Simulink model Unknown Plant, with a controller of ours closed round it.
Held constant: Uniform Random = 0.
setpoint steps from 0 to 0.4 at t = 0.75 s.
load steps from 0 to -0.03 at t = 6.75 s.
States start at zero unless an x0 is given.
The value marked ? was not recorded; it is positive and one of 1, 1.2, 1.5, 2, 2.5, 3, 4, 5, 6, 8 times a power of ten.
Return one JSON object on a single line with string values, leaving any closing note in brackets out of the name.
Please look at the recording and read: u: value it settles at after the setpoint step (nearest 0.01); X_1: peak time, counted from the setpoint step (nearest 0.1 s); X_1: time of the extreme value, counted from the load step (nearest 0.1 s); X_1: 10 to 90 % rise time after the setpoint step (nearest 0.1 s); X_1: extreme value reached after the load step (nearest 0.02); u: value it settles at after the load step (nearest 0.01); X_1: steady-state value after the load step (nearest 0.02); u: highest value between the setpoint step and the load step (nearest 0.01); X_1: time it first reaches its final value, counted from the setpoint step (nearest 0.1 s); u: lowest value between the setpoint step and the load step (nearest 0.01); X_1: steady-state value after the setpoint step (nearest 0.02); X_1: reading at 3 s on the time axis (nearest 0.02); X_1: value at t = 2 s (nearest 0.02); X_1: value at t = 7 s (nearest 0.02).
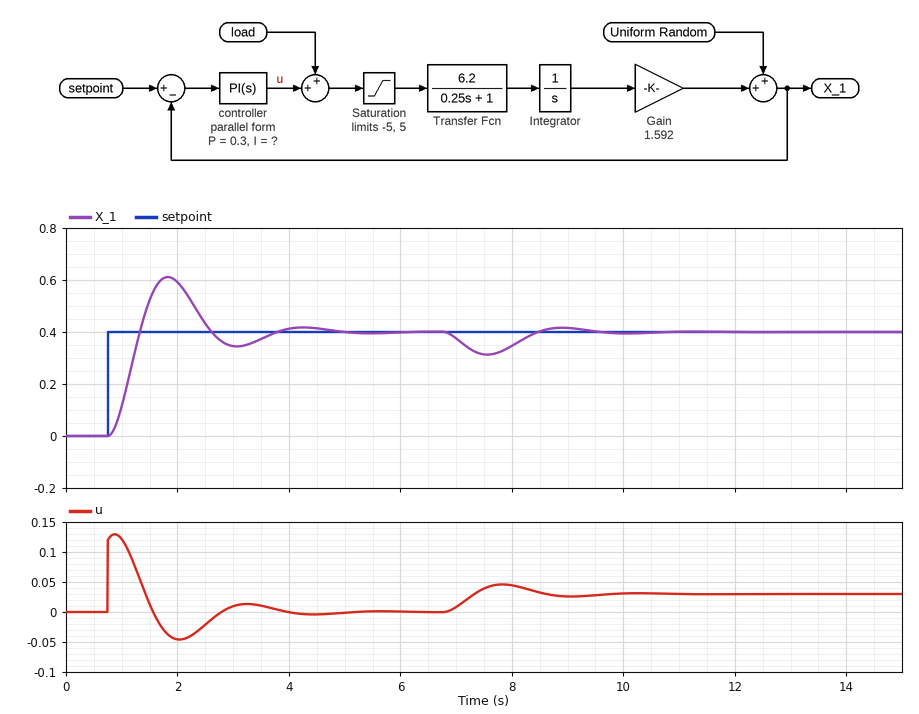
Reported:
{"u: value it settles at after the setpoint step": "0.00", "X_1: peak time, counted from the setpoint step": "1.1 s", "X_1: time of the extreme value, counted from the load step": "0.8 s", "X_1: 10 to 90 % rise time after the setpoint step": "0.4 s", "X_1: extreme value reached after the load step": "0.32", "u: value it settles at after the load step": "0.03", "X_1: steady-state value after the load step": "0.40", "u: highest value between the setpoint step and the load step": "0.13", "X_1: time it first reaches its final value, counted from the setpoint step": "0.6 s", "u: lowest value between the setpoint step and the load step": "-0.05", "X_1: steady-state value after the setpoint step": "0.40", "X_1: reading at 3 s on the time axis": "0.34", "X_1: value at t = 2 s": "0.60", "X_1: value at t = 7 s": "0.38"}
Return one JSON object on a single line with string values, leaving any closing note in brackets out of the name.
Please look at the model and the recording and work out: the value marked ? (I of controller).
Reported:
{"the value marked ?": "0.4"}
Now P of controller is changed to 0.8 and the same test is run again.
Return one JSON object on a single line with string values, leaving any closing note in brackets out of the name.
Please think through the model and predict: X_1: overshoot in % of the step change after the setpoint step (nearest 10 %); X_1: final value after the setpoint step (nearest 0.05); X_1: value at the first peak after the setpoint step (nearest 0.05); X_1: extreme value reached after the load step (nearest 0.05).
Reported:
{"X_1: overshoot in % of the step change after the setpoint step": "40 %", "X_1: final value after the setpoint step": "0.40", "X_1: value at the first peak after the setpoint step": "0.55", "X_1: extreme value reached after the load step": "0.35"}
